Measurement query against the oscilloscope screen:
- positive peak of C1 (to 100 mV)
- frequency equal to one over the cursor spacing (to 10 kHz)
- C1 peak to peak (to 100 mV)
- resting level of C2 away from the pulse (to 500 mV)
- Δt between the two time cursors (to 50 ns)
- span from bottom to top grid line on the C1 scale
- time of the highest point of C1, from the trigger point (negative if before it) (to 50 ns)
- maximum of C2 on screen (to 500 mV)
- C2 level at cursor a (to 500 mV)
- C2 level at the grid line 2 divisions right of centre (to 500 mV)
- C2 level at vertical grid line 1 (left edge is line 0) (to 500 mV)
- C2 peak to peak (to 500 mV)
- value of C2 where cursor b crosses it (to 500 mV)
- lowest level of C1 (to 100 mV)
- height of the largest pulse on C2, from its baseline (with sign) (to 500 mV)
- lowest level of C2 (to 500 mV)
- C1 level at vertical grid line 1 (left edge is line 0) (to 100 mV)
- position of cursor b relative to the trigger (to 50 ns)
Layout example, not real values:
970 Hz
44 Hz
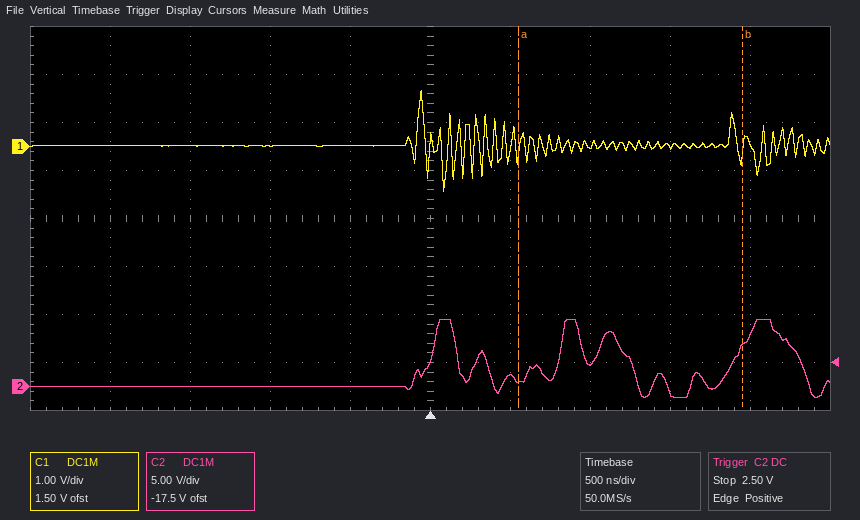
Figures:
1.2 V
710 kHz
2.1 V
0.0 V
1.40 µs
8 V
-50 ns
7.0 V
500 mV
2.5 V
0.0 V
8.0 V
4.0 V
-900 mV
+7.0 V
-1.0 V
0.0 V
+1.95 µs
